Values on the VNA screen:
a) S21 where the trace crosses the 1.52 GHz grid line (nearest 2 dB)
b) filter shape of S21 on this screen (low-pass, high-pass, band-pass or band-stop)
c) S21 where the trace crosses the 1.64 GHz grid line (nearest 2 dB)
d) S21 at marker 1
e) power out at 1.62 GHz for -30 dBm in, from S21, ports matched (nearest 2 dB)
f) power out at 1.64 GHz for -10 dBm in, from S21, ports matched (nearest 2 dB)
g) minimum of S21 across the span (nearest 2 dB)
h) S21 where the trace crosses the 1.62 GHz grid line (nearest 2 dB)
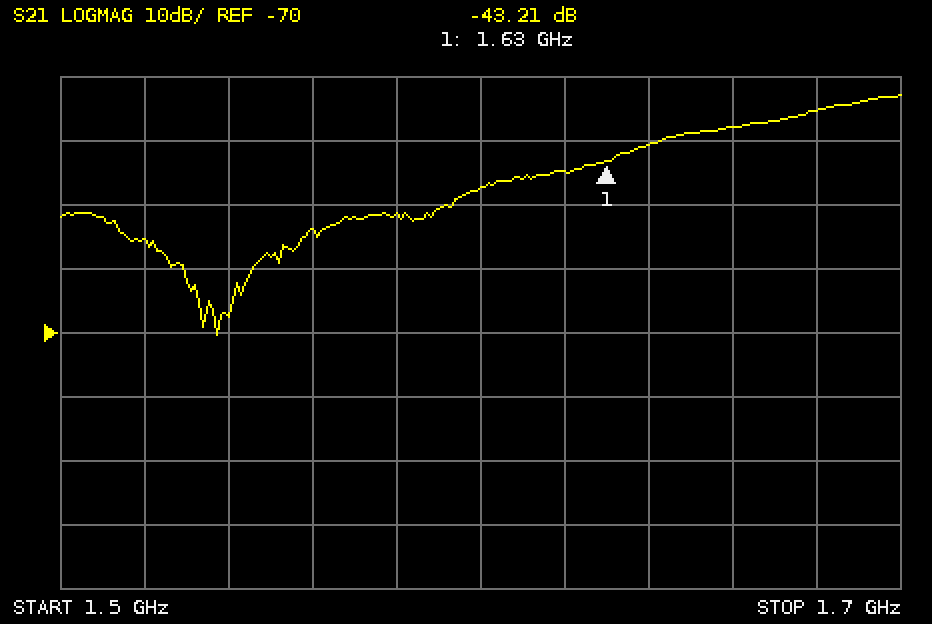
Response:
-56 dB
high-pass
-40 dB
-43.21 dB
-74 dBm
-50 dBm
-70 dB
-44 dB
